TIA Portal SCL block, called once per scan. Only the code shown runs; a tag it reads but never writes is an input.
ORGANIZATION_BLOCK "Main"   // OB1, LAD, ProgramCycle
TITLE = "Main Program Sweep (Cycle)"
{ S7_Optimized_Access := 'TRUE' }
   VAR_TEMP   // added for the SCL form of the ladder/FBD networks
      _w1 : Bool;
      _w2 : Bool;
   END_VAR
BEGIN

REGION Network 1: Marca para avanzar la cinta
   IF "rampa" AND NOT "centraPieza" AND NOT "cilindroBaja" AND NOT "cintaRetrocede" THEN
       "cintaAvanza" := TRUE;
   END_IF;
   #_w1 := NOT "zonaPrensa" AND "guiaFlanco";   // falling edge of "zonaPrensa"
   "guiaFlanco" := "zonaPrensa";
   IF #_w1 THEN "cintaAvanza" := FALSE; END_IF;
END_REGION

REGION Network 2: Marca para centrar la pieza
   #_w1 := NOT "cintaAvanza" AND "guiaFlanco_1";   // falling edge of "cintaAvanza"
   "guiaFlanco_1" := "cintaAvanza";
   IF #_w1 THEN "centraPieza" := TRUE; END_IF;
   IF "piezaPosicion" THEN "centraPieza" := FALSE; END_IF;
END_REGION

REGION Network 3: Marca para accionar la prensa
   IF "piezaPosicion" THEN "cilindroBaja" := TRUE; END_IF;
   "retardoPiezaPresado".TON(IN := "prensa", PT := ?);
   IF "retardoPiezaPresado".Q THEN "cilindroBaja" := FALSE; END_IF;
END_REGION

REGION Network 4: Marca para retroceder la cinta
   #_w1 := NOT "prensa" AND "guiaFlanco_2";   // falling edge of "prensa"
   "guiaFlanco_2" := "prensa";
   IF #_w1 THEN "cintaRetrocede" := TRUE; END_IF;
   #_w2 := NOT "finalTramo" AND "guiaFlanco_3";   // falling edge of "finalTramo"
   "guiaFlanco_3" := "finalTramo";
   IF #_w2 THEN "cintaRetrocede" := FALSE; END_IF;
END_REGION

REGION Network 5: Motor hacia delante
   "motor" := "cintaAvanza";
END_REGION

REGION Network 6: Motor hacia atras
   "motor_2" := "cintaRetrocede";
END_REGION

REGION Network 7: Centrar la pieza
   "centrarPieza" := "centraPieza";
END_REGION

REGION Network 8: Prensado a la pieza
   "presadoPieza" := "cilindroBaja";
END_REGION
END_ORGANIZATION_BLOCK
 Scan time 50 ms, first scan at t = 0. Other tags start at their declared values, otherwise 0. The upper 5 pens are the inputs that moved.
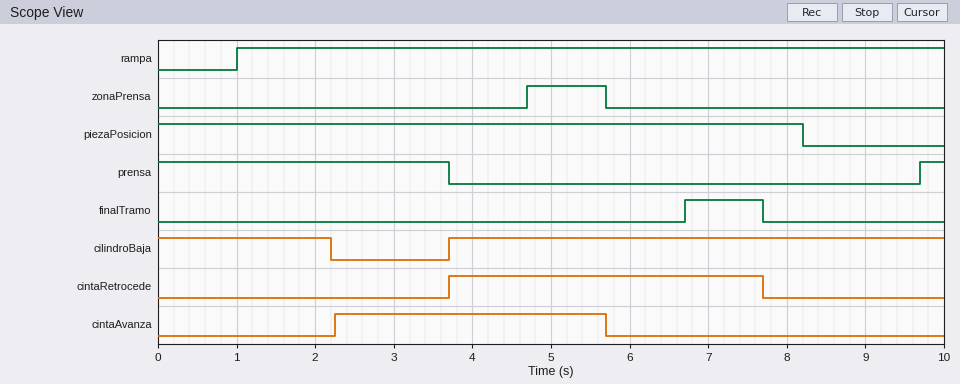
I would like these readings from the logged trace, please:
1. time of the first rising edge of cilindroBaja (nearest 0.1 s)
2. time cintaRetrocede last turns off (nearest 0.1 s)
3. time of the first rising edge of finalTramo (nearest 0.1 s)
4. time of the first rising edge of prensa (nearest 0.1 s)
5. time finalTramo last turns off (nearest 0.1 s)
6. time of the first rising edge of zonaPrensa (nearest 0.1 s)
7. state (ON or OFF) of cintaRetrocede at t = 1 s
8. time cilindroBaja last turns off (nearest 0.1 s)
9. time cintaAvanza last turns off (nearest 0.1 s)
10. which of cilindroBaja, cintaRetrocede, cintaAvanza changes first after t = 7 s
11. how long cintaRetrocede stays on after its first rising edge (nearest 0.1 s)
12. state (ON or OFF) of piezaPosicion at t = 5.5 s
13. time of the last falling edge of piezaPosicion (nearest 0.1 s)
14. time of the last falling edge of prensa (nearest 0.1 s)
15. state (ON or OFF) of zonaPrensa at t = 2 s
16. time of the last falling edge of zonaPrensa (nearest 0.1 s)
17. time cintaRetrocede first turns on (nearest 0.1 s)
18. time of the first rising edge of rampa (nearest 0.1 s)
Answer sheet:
3.7 s
7.7 s
6.7 s
9.7 s
7.7 s
4.7 s
OFF
2.2 s
5.7 s
cintaRetrocede
4.0 s
ON
8.2 s
3.7 s
OFF
5.7 s
3.7 s
1.0 s
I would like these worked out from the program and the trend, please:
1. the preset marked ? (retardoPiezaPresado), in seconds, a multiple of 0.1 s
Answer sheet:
2.2 s
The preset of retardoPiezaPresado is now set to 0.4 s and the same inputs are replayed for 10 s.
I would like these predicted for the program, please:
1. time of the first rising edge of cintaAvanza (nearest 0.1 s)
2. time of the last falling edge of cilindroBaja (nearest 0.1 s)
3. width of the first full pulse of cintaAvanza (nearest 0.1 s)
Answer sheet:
1.0 s
0.4 s
4.7 s
